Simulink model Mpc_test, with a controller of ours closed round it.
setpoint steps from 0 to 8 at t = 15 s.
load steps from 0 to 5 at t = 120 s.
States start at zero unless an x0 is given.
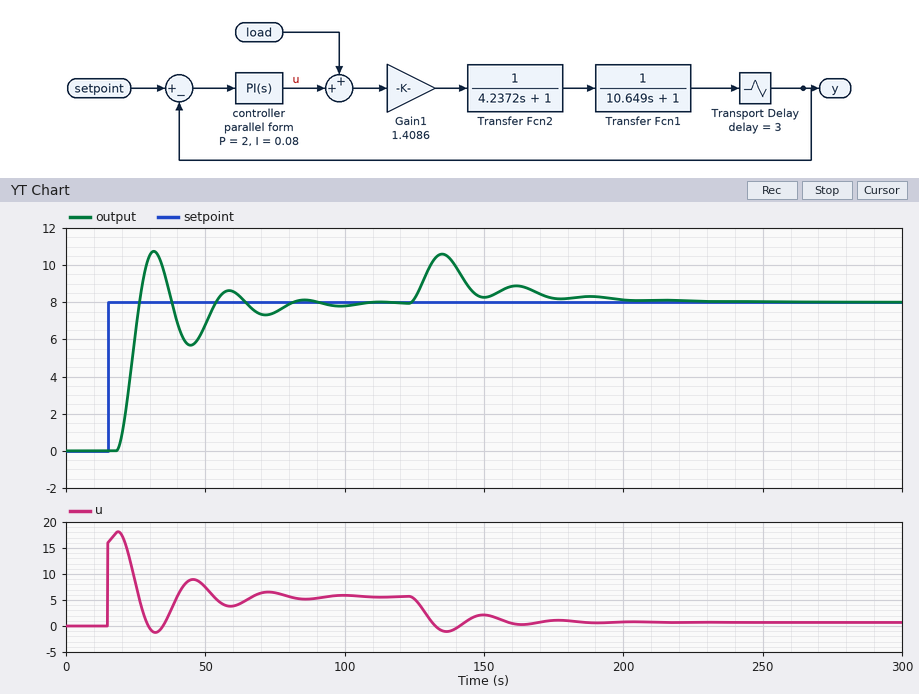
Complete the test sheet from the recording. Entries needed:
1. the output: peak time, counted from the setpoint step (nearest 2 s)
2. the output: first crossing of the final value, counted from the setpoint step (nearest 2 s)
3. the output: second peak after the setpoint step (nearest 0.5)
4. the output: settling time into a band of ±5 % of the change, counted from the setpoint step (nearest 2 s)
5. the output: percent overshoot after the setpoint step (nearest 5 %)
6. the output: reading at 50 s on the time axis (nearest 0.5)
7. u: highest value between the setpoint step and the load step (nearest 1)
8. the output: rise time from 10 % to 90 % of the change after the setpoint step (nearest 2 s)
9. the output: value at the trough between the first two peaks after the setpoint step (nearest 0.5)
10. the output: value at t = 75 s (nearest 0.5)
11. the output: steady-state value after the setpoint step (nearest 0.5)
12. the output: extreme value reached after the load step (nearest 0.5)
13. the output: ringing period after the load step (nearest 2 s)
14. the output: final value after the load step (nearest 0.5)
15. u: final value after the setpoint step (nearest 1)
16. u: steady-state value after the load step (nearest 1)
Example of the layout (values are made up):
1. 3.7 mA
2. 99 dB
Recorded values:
1. 16 s
2. 12 s
3. 8.5
4. 62 s
5. 35 %
6. 7.0
7. 18
8. 6 s
9. 5.5
10. 7.5
11. 8.0
12. 10.5
13. 26 s
14. 8.0
15. 6
16. 1
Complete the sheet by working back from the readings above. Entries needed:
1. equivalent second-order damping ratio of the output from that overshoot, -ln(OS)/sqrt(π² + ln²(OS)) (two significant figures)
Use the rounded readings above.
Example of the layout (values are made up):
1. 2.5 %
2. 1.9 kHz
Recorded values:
1. 0.32
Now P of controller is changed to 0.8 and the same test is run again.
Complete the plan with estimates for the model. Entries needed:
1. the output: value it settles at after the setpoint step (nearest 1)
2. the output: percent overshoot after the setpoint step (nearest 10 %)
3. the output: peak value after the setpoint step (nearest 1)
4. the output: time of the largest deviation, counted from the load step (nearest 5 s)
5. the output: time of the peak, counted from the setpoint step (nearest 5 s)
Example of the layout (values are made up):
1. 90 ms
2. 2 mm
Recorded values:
1. 8
2. 20 %
3. 10
4. 20 s
5. 25 s
